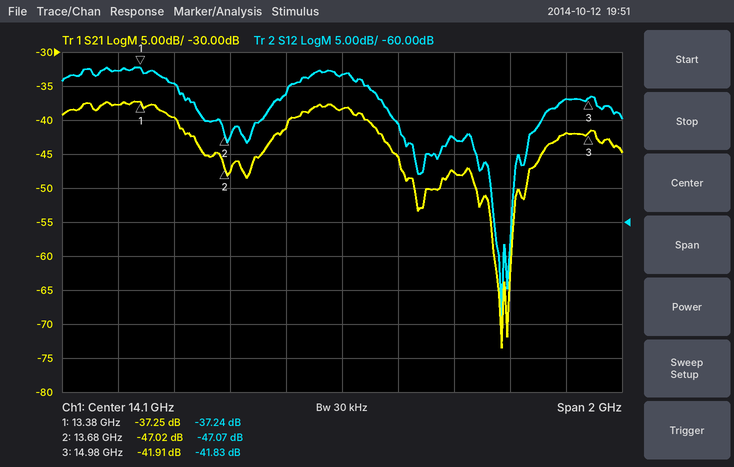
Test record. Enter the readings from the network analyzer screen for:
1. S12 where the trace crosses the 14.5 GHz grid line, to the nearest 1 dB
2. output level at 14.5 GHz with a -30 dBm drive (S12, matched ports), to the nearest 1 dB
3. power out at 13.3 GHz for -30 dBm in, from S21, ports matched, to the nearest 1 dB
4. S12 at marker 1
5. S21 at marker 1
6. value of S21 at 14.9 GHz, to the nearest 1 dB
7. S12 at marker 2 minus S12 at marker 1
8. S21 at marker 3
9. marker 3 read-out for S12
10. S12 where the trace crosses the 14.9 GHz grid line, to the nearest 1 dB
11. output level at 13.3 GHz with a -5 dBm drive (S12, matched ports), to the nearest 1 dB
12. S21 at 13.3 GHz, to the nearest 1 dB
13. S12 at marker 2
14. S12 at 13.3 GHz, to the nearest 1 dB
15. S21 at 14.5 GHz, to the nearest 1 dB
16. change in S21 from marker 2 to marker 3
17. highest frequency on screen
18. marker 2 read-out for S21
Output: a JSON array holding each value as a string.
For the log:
["-48 dB", "-78 dBm", "-68 dBm", "-37.24 dB", "-37.25 dB", "-42 dB", "-9.83 dB", "-41.91 dB", "-41.83 dB", "-42 dB", "-43 dBm", "-38 dB", "-47.07 dB", "-38 dB", "-48 dB", "5.11 dB", "15.1 GHz", "-47.02 dB"]
